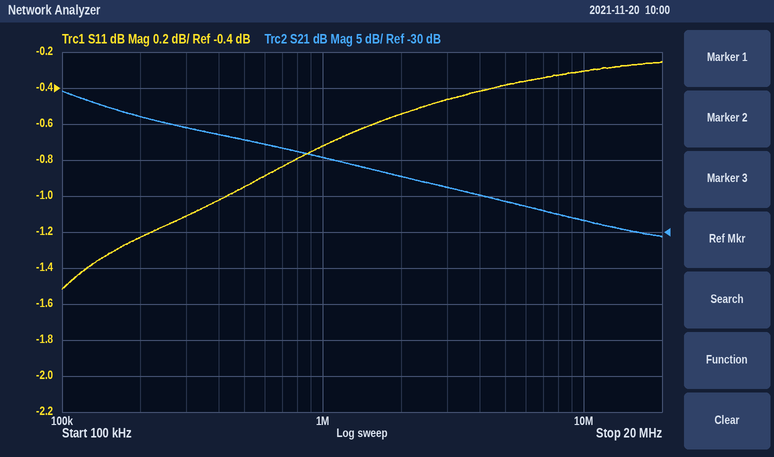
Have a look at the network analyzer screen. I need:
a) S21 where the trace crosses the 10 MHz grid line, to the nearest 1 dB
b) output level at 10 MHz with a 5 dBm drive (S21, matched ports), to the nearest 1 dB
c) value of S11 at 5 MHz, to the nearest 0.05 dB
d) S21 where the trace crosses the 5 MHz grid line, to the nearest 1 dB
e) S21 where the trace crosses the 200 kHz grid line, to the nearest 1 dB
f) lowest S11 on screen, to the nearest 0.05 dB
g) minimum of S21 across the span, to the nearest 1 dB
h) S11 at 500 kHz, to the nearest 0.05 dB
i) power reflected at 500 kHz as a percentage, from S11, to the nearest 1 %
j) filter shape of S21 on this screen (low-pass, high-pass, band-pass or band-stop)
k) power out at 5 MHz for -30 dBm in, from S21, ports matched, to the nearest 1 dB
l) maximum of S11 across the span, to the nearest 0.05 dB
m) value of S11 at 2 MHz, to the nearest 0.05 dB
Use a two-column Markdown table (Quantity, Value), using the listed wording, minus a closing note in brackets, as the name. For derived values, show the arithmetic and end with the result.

| Quantity | Value |
|---|---|
| S21 where the trace crosses the 10 MHz grid line, to the nearest 1 dB | -28 dB |
| output level at 10 MHz with a 5 dBm drive (S21, matched ports), to the nearest 1 dB | 5 dBm + (-28 dB) = -23 dBm |
| value of S11 at 5 MHz, to the nearest 0.05 dB | -0.40 dB |
| S21 where the trace crosses the 5 MHz grid line, to the nearest 1 dB | -26 dB |
| S21 where the trace crosses the 200 kHz grid line, to the nearest 1 dB | -14 dB |
| lowest S11 on screen, to the nearest 0.05 dB | -1.50 dB |
| minimum of S21 across the span, to the nearest 1 dB | -31 dB |
| S11 at 500 kHz, to the nearest 0.05 dB | -0.95 dB |
| power reflected at 500 kHz as a percentage, from S11, to the nearest 1 % | 10^(-0.95/10) ≈ 80 % |
| filter shape of S21 on this screen | low-pass |
| power out at 5 MHz for -30 dBm in, from S21, ports matched, to the nearest 1 dB | -30 dBm + (-26 dB) = -56 dBm |
| maximum of S11 across the span, to the nearest 0.05 dB | -0.25 dB |
| value of S11 at 2 MHz, to the nearest 0.05 dB | -0.55 dB |
